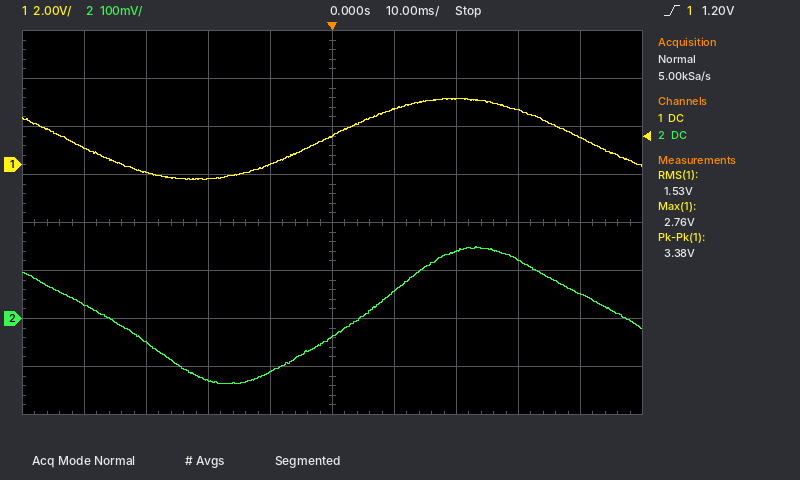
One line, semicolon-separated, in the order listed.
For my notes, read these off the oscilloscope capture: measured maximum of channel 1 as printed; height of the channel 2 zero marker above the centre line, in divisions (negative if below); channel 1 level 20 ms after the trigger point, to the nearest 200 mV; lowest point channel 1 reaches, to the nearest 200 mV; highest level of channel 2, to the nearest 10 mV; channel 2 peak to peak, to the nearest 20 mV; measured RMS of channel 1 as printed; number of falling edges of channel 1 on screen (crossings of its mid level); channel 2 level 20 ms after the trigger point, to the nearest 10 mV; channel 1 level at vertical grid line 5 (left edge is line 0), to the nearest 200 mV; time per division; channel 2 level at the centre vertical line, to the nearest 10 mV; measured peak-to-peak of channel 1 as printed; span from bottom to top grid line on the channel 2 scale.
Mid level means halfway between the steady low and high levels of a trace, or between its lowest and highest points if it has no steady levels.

2.76 V; -2.0 div; 2.8 V; -600 mV; 150 mV; 280 mV; 1.53 V; 2; 140 mV; 1.2 V; 10 ms; -40 mV; 3.38 V; 800 mV
